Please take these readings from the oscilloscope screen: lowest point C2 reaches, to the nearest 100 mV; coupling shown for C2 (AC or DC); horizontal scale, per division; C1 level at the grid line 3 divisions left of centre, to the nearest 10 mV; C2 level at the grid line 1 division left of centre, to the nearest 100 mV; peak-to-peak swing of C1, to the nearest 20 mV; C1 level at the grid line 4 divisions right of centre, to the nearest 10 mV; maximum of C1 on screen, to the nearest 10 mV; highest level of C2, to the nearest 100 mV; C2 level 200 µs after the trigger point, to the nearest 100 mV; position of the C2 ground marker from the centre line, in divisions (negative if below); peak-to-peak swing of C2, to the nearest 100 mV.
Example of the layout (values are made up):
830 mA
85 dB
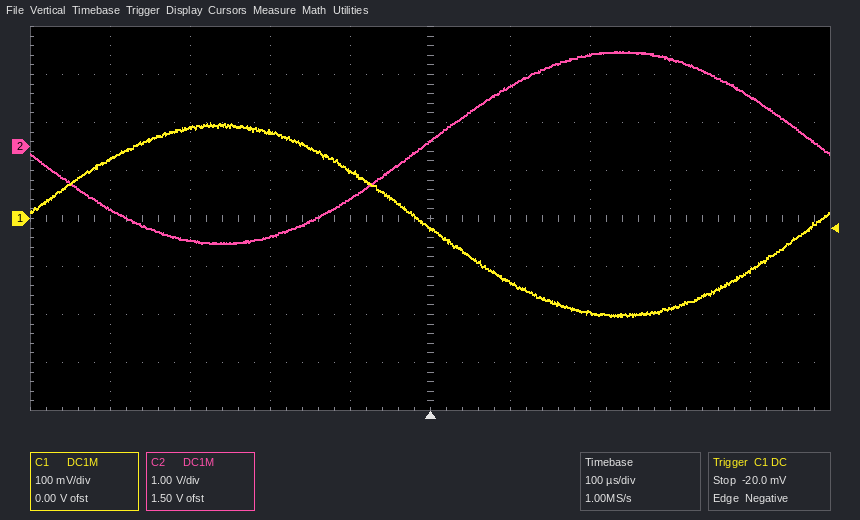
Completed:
-2.0 V
DC
100 µs
190 mV
-1.1 V
400 mV
-110 mV
200 mV
2.0 V
1.9 V
+1.5 div
4.0 V
